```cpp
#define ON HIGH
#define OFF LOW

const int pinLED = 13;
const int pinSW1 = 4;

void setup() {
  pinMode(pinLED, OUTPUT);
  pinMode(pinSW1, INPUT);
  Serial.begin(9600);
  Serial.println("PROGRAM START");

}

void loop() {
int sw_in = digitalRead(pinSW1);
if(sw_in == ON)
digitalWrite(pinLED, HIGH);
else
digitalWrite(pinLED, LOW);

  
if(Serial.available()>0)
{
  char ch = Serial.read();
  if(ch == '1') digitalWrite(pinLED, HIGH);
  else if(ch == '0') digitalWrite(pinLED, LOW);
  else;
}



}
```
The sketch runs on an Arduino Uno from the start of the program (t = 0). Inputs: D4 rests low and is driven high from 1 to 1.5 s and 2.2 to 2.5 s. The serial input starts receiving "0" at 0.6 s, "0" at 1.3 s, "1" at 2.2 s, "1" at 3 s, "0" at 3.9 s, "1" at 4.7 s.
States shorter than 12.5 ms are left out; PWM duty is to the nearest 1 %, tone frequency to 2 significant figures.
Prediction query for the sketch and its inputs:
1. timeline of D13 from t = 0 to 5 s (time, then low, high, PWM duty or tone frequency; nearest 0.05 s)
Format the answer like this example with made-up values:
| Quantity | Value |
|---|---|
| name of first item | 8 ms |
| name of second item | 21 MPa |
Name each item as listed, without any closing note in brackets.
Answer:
| Quantity | Value |
|---|---|
| timeline of D13 from t = 0 to 5 s | 0 s low; 1 s high; 1.5 s low; 2.2 s high; 2.5 s low |
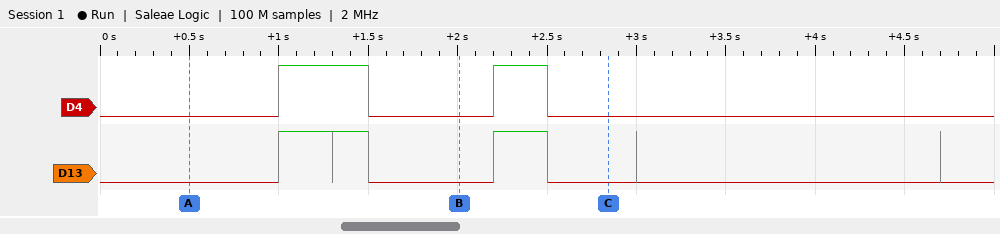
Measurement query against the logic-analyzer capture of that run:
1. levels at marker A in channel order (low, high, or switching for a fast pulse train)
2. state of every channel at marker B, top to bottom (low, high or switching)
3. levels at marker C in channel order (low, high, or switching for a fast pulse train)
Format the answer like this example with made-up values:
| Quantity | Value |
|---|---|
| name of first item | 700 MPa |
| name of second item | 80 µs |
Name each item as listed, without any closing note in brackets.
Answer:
| Quantity | Value |
|---|---|
| levels at marker A in channel order | D4 low, D13 low |
| state of every channel at marker B, top to bottom | D4 low, D13 low |
| levels at marker C in channel order | D4 low, D13 low |
